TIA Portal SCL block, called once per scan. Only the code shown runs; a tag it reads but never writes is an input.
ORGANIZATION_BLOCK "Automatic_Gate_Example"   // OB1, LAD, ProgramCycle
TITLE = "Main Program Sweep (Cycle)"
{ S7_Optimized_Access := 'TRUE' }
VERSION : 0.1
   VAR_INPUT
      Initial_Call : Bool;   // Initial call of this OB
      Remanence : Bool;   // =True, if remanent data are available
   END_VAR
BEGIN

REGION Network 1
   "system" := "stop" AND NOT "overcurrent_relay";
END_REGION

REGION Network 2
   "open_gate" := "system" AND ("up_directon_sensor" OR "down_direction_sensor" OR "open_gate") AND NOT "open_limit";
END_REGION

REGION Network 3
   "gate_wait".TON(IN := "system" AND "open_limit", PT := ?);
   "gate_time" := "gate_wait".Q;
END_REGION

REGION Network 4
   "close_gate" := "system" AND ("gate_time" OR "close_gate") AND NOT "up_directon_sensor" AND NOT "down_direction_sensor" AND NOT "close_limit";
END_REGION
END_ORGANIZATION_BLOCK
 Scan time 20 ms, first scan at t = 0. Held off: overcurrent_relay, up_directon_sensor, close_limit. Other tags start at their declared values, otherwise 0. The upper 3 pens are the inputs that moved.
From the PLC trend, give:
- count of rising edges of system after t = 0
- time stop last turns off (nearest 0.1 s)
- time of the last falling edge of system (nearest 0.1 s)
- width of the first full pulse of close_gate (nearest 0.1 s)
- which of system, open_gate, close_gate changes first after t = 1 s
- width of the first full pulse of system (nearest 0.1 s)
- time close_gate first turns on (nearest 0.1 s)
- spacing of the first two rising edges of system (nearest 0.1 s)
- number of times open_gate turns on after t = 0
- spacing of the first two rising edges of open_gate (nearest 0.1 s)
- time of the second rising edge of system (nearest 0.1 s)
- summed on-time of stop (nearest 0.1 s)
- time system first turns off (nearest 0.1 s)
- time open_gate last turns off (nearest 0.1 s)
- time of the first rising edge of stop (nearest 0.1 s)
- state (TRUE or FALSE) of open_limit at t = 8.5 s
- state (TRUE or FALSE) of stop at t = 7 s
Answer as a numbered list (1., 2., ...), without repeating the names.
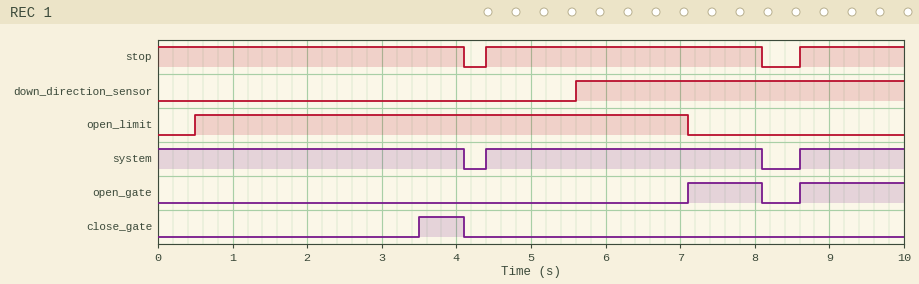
1. 2
2. 8.1 s
3. 8.1 s
4. 0.6 s
5. close_gate
6. 3.7 s
7. 3.5 s
8. 4.2 s
9. 2
10. 1.5 s
11. 8.6 s
12. 9.2 s
13. 4.1 s
14. 8.1 s
15. 4.4 s
16. FALSE
17. TRUE
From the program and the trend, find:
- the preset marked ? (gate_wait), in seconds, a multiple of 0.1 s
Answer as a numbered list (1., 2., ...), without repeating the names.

1. 3.0 s
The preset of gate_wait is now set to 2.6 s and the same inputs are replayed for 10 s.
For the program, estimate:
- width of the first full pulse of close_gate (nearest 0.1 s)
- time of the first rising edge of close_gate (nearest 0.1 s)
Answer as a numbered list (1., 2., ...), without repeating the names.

1. 1.0 s
2. 3.1 s
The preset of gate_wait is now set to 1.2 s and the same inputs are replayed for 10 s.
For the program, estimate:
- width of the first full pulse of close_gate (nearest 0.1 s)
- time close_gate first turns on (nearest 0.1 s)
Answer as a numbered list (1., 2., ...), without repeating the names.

1. 2.4 s
2. 1.7 s
